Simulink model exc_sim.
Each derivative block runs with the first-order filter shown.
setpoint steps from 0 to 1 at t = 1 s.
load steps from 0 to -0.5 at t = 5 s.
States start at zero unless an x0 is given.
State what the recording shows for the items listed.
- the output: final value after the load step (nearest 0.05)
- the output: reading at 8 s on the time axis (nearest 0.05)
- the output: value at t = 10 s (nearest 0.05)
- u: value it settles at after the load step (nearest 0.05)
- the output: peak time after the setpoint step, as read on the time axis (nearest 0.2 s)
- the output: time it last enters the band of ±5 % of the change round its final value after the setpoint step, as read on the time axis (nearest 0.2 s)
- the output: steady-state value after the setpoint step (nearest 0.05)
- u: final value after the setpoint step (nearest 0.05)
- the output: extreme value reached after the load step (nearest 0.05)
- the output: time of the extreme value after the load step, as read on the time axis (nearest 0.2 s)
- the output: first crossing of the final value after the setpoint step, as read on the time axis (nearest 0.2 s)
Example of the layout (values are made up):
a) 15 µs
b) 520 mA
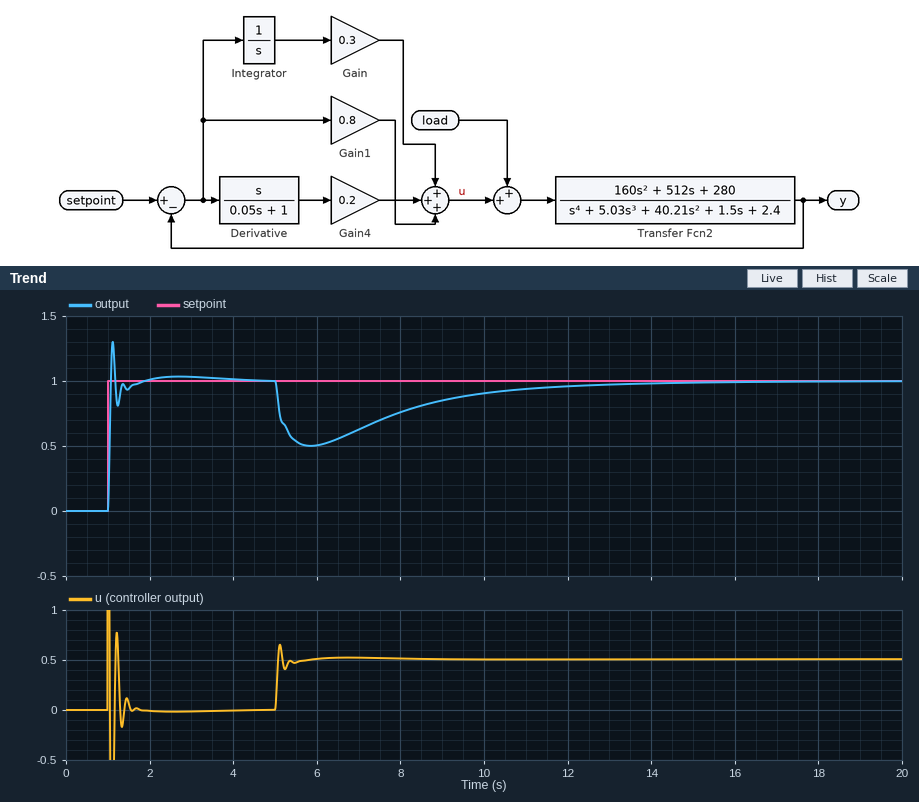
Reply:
a) 1.00
b) 0.75
c) 0.90
d) 0.50
e) 1.2 s
f) 1.6 s
g) 1.00
h) 0.00
i) 0.50
j) 5.8 s
k) 1.0 s
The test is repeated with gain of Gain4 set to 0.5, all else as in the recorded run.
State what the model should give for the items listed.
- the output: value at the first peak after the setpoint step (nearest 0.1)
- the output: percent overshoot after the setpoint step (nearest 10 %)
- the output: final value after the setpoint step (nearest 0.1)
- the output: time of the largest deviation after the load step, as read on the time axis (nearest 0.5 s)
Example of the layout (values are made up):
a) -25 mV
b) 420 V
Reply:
a) 1.4
b) 40 %
c) 1.0
d) 6.5 s
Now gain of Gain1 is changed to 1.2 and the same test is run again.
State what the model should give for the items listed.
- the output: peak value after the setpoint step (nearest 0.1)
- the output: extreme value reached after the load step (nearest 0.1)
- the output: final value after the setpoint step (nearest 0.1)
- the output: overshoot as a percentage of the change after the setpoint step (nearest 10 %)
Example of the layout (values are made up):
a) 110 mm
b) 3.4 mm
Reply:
a) 1.4
b) 0.6
c) 1.0
d) 40 %
